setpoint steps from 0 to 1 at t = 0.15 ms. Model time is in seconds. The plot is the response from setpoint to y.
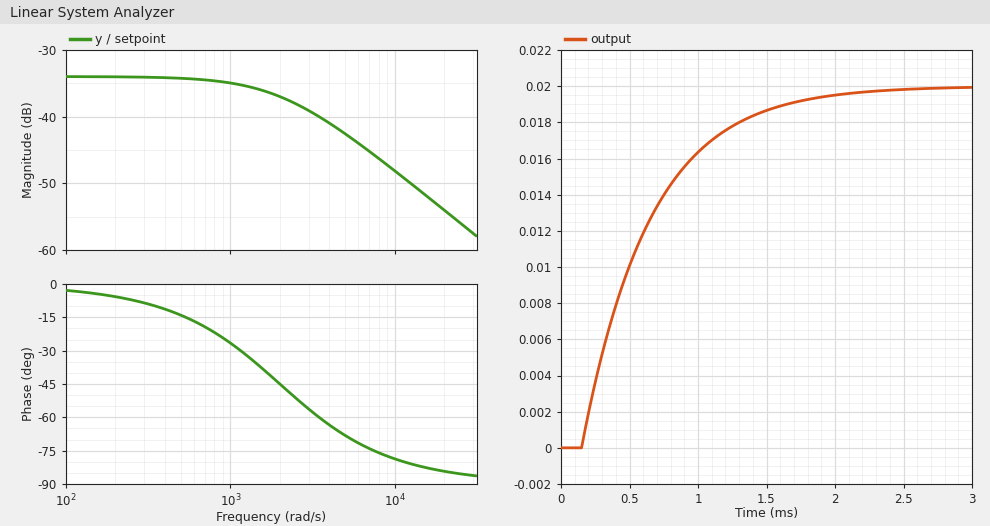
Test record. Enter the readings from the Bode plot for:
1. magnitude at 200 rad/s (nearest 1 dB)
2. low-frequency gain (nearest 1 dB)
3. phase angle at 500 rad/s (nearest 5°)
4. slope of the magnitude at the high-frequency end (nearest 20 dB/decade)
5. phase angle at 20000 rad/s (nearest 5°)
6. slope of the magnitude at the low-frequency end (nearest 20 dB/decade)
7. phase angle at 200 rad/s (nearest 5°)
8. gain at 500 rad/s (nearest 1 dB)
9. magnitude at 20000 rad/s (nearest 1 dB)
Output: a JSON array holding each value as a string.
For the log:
["-34 dB", "-34 dB", "-15°", "-20 dB/decade", "-85°", "0 dB/decade", "-5°", "-34 dB", "-54 dB"]
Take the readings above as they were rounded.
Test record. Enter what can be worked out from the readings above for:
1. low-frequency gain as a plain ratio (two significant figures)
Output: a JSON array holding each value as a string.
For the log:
["0.020"]
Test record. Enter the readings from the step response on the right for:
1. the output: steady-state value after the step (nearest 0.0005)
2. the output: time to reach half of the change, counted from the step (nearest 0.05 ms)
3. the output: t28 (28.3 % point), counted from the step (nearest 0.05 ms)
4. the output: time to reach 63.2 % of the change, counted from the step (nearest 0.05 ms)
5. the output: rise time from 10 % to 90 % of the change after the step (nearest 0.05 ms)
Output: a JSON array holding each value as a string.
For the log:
["0.0200", "0.35 ms", "0.15 ms", "0.50 ms", "1.10 ms"]
